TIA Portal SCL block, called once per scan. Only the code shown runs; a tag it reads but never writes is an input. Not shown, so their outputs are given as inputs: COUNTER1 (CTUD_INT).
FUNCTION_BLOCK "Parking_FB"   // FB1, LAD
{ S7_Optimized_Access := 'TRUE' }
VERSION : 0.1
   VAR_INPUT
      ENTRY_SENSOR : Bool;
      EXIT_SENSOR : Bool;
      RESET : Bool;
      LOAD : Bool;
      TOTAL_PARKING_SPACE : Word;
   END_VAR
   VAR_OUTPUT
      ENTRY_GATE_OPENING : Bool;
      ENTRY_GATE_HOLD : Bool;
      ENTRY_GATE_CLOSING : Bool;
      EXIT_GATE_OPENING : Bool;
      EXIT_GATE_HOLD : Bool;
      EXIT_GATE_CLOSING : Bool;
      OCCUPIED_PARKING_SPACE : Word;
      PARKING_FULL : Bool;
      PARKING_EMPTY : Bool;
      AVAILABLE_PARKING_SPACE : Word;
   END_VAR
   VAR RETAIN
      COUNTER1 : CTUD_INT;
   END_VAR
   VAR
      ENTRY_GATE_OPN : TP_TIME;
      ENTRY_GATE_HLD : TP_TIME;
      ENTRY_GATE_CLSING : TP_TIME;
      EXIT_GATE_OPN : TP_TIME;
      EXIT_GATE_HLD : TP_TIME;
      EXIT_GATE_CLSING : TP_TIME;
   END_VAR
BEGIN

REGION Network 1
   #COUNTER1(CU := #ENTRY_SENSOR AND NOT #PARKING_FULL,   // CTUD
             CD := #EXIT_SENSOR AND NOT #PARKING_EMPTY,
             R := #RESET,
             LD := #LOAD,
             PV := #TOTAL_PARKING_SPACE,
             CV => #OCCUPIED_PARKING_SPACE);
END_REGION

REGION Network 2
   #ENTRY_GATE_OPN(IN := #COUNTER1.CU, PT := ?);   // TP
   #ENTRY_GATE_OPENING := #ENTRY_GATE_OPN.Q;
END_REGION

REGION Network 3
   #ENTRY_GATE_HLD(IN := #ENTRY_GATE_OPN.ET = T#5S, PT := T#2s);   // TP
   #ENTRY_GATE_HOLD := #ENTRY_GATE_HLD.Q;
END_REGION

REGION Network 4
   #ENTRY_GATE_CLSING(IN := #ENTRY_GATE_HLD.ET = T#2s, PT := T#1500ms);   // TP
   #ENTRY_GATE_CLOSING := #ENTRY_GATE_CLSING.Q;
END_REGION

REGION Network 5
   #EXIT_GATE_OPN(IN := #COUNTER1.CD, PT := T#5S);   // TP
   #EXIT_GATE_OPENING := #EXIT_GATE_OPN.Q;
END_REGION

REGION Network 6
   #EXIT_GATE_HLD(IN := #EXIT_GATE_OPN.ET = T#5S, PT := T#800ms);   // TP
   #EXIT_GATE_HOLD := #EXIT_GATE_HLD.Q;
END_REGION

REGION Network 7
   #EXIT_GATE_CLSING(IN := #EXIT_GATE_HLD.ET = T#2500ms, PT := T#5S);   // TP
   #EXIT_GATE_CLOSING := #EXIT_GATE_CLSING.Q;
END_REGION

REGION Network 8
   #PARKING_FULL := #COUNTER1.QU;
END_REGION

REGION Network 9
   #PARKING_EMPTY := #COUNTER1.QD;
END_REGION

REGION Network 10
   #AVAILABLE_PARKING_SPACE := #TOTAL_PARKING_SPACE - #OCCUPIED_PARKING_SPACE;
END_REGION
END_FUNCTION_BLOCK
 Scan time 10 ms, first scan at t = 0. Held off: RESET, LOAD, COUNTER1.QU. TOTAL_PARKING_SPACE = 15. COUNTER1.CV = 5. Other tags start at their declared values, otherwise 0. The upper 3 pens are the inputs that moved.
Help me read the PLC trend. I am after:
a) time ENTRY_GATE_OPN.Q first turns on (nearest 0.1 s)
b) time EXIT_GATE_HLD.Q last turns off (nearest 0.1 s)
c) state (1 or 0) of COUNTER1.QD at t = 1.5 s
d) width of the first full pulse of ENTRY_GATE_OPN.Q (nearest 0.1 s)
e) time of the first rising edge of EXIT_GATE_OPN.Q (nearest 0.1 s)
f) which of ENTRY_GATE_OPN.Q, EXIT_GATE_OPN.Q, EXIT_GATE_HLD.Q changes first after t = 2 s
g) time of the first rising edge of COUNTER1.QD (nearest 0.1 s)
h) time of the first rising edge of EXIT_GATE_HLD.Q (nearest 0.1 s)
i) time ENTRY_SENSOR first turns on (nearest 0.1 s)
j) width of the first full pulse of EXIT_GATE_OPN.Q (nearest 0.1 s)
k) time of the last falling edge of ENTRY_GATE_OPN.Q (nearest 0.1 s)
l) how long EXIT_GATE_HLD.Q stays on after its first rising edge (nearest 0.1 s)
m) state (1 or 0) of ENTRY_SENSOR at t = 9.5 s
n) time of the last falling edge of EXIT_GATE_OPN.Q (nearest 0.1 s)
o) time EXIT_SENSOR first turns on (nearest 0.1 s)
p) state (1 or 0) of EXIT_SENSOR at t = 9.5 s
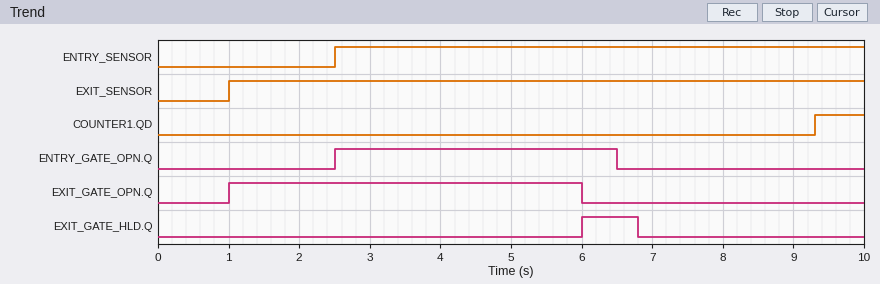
2.5 s
6.8 s
0
4.0 s
1.0 s
ENTRY_GATE_OPN.Q
9.3 s
6.0 s
2.5 s
5.0 s
6.5 s
0.8 s
1
6.0 s
1.0 s
1
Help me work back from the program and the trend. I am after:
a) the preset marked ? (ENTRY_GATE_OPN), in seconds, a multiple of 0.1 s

4.0 s
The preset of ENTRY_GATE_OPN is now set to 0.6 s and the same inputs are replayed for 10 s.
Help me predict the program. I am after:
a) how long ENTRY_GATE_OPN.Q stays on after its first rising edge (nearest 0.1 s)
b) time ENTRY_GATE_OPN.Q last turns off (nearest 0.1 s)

0.6 s
3.1 s
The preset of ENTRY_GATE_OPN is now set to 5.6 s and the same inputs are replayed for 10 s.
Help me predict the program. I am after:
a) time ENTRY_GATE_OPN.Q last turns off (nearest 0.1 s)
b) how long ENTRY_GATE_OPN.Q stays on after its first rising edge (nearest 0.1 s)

8.1 s
5.6 s
